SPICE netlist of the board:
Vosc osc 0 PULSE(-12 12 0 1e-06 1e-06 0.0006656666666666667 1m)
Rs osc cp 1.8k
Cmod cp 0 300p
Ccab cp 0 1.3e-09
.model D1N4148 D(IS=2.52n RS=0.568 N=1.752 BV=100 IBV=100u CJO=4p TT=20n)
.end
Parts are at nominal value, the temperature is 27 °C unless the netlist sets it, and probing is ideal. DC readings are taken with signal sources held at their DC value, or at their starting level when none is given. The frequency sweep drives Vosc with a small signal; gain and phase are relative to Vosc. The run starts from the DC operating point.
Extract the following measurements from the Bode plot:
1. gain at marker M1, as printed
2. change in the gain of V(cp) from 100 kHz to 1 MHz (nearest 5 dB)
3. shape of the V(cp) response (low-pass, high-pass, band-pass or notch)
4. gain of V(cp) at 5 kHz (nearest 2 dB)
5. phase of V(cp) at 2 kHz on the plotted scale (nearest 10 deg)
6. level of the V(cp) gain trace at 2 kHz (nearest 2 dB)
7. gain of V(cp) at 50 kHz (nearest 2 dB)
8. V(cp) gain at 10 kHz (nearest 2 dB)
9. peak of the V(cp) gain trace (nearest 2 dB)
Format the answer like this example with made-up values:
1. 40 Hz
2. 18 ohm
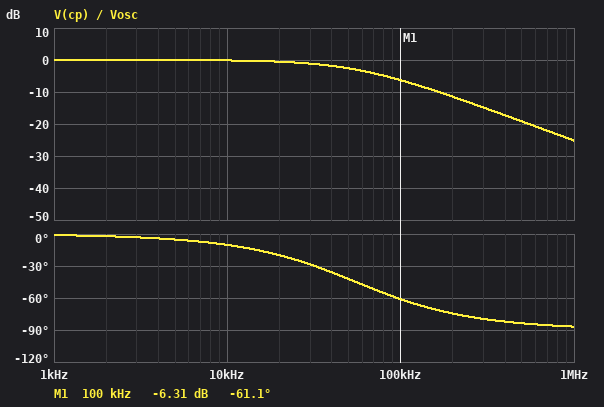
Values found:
1. -6.31 dB
2. -20 dB
3. low-pass
4. 0 dB
5. 0 deg
6. 0 dB
7. -2 dB
8. 0 dB
9. 0 dB
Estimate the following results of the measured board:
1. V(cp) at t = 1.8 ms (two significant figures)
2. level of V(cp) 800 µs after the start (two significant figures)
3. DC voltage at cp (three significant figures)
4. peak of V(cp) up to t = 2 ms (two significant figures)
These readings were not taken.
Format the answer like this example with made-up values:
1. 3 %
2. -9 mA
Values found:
1. -12 V
2. -12 V
3. -12.0 V
4. 12 V
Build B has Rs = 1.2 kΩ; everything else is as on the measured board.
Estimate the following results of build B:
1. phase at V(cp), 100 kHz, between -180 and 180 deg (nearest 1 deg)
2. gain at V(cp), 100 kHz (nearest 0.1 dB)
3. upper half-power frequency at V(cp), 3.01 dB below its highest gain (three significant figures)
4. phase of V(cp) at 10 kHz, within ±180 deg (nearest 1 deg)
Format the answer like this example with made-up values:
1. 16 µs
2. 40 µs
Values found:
1. -50 deg
2. -3.9 dB
3. 82.9 kHz
4. -7 deg
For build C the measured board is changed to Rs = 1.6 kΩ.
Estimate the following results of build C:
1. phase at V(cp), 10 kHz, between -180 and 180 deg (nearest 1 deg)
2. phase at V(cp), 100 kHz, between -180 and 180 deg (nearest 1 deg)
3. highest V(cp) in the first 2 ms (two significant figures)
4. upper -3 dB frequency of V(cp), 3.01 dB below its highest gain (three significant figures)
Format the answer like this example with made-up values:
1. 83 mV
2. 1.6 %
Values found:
1. -9 deg
2. -58 deg
3. 12 V
4. 62.2 kHz
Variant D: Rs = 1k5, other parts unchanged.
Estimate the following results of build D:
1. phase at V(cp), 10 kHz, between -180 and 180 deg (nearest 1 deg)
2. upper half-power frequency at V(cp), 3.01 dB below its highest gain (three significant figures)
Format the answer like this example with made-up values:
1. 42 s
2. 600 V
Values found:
1. -9 deg
2. 66.3 kHz
